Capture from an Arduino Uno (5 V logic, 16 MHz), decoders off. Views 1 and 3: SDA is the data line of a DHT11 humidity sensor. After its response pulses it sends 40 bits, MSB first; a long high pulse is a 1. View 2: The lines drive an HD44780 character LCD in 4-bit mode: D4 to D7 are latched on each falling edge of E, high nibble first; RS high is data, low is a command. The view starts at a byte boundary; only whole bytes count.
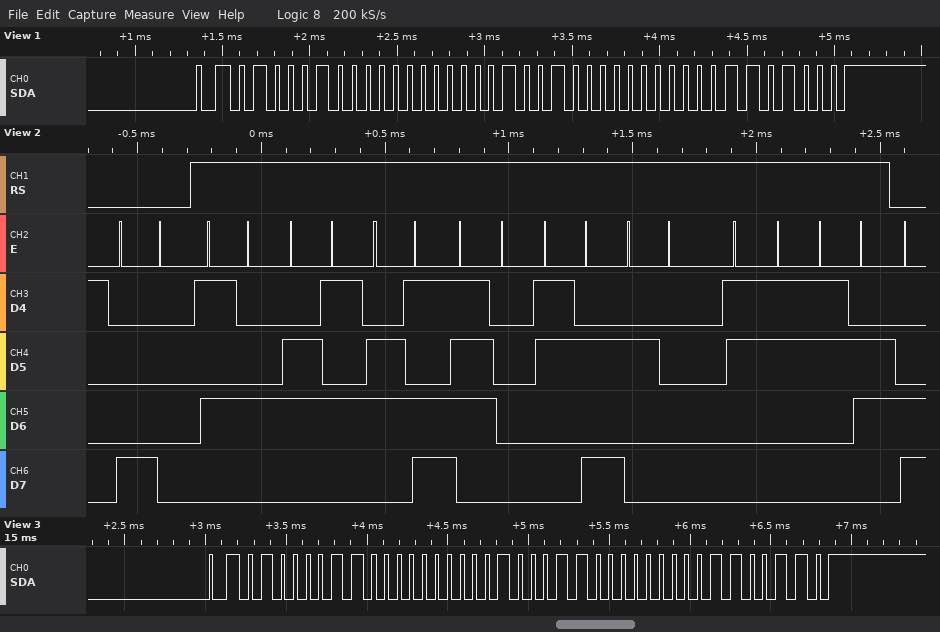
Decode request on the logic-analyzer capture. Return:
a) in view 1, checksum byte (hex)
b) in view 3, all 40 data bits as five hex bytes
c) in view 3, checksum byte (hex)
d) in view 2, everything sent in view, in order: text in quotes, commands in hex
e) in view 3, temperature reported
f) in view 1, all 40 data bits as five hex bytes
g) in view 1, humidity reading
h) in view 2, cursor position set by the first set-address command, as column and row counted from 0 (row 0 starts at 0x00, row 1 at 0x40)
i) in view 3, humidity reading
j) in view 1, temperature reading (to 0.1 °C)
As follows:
0x68
43 00 23 00 66
0x66
0x80 "Temp: 36"
35.0 °C
44 00 24 00 68
68 %
column 0, row 0
67 %
36.0 °C
